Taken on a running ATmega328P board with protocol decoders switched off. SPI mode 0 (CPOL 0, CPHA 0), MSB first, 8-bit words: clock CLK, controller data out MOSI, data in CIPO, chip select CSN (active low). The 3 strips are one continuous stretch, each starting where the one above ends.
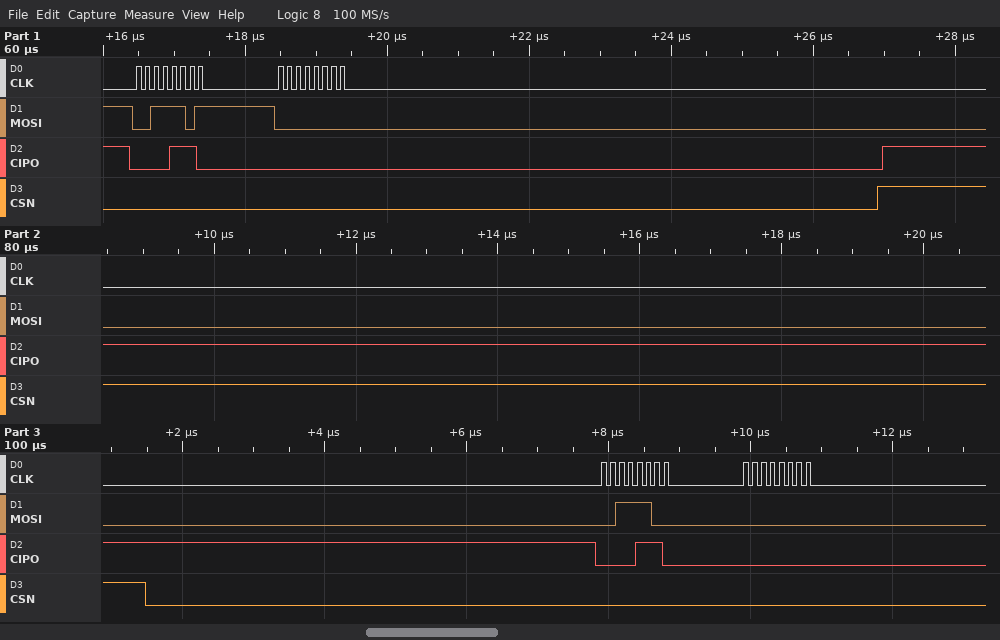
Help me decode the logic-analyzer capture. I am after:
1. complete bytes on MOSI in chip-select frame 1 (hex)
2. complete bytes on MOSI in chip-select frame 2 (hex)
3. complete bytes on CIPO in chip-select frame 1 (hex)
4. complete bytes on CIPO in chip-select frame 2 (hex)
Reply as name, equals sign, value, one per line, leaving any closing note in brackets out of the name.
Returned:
complete bytes on MOSI in chip-select frame 1 = 0x3D 0x00
complete bytes on MOSI in chip-select frame 2 = 0x3C 0x00
complete bytes on CIPO in chip-select frame 1 = 0x0E 0x00
complete bytes on CIPO in chip-select frame 2 = 0x0E 0x00
